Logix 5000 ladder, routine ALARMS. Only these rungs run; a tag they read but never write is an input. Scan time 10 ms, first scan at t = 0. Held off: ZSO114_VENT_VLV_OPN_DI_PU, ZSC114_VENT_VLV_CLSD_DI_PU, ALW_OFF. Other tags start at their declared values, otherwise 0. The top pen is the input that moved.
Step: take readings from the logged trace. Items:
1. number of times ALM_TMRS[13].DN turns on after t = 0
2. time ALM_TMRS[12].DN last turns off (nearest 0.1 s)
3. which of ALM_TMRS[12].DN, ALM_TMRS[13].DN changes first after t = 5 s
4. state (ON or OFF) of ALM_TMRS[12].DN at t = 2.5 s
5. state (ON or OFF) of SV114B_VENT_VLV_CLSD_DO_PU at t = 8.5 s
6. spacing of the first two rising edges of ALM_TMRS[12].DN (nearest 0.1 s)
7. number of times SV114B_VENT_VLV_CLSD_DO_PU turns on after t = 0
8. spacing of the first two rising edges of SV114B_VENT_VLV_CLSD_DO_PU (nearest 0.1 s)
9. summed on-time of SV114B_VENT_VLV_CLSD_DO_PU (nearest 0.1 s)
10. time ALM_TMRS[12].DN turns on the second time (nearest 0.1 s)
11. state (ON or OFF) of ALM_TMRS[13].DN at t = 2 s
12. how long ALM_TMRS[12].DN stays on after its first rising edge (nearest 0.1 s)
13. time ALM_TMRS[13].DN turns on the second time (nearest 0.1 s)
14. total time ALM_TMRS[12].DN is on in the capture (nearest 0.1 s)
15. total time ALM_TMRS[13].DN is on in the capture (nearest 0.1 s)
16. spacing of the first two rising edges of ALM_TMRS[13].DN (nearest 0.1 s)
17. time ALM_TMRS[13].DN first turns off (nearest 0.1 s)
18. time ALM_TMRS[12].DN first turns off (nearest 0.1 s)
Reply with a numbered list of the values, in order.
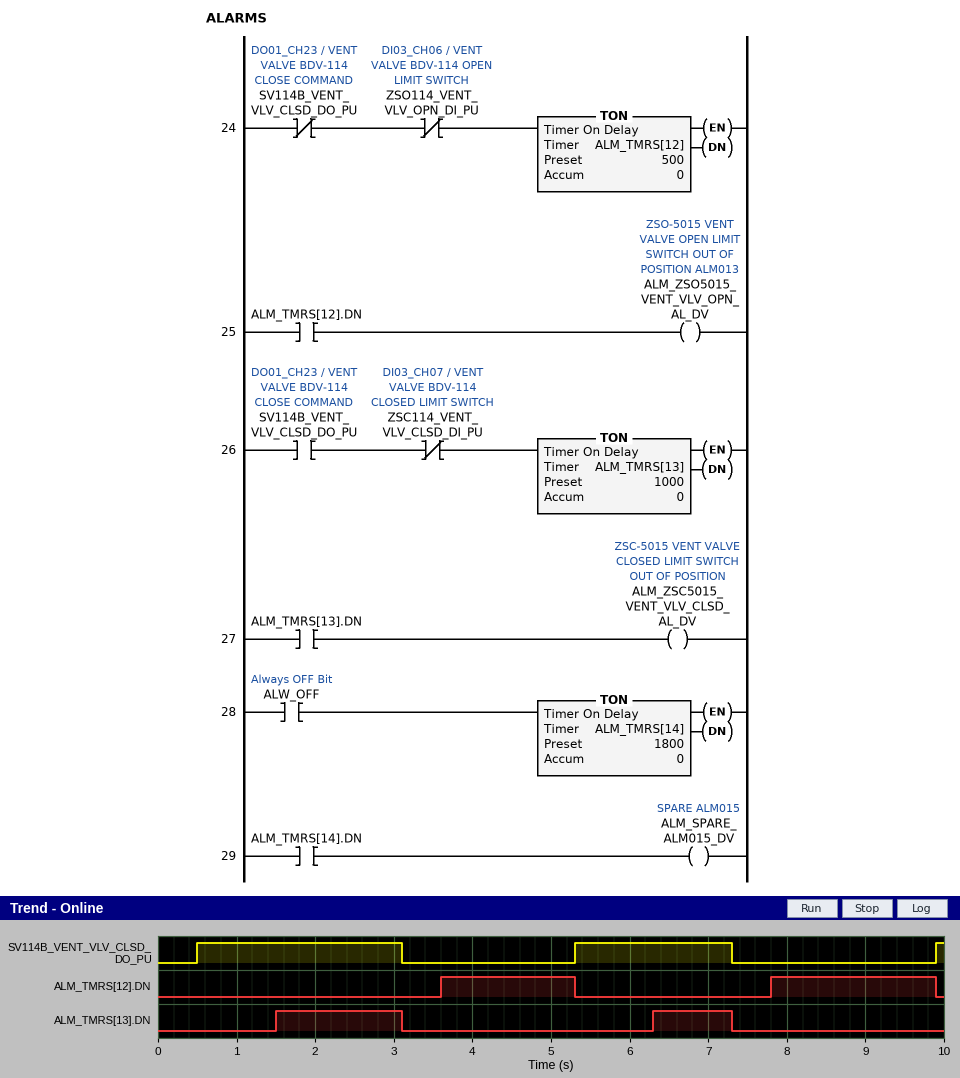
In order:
1. 2
2. 9.9 s
3. ALM_TMRS[12].DN
4. OFF
5. OFF
6. 4.2 s
7. 3
8. 4.8 s
9. 4.7 s
10. 7.8 s
11. ON
12. 1.7 s
13. 6.3 s
14. 3.8 s
15. 2.6 s
16. 4.8 s
17. 3.1 s
18. 5.3 s
